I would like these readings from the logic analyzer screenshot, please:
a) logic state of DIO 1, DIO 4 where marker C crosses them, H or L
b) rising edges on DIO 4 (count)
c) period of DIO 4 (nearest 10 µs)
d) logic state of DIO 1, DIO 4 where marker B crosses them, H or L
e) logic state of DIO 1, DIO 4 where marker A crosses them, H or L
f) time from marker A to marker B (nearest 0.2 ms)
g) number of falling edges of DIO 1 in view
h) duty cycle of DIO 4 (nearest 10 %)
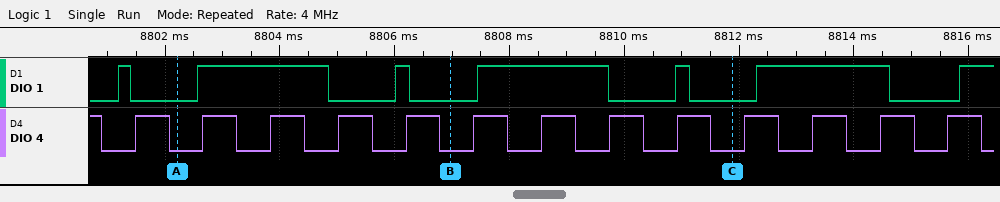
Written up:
DIO 1=L, DIO 4=L
13
1180 µs
DIO 1=L, DIO 4=L
DIO 1=L, DIO 4=L
4.8 ms
6
50 %
